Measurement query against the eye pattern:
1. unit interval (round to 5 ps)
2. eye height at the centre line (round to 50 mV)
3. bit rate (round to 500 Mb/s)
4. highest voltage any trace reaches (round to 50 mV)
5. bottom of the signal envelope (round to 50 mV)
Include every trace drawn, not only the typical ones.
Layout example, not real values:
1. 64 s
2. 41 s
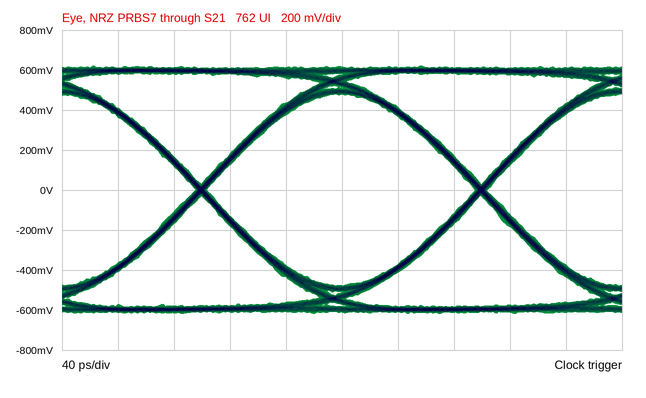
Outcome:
1. 200 ps
2. 950 mV
3. 5.0 Gb/s
4. 600 mV
5. -600 mV
